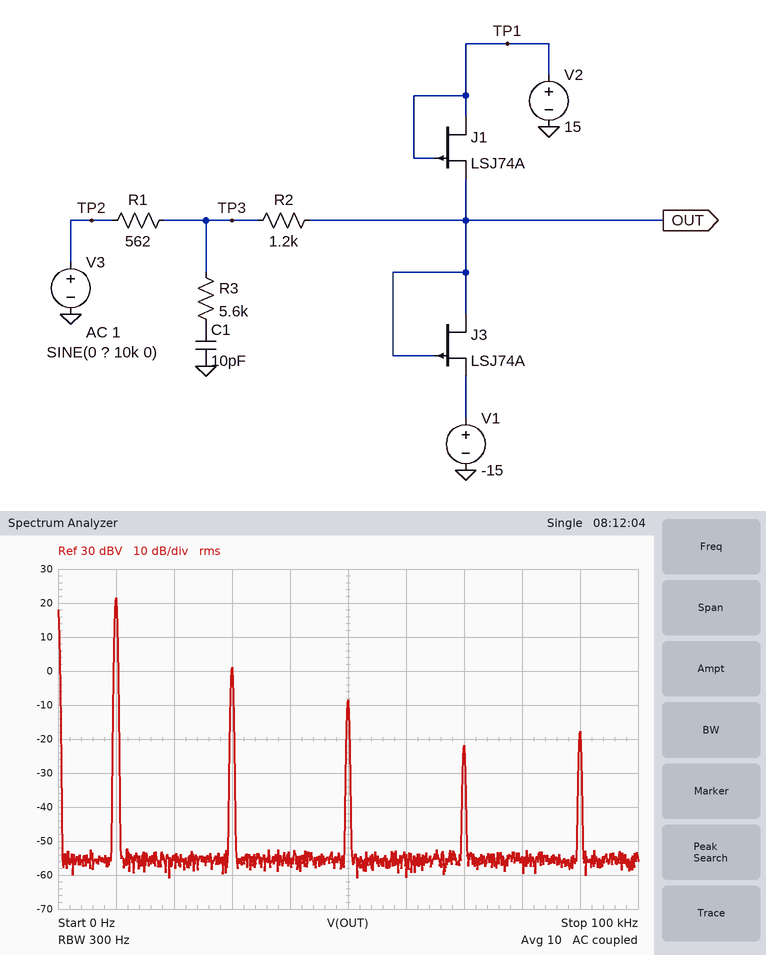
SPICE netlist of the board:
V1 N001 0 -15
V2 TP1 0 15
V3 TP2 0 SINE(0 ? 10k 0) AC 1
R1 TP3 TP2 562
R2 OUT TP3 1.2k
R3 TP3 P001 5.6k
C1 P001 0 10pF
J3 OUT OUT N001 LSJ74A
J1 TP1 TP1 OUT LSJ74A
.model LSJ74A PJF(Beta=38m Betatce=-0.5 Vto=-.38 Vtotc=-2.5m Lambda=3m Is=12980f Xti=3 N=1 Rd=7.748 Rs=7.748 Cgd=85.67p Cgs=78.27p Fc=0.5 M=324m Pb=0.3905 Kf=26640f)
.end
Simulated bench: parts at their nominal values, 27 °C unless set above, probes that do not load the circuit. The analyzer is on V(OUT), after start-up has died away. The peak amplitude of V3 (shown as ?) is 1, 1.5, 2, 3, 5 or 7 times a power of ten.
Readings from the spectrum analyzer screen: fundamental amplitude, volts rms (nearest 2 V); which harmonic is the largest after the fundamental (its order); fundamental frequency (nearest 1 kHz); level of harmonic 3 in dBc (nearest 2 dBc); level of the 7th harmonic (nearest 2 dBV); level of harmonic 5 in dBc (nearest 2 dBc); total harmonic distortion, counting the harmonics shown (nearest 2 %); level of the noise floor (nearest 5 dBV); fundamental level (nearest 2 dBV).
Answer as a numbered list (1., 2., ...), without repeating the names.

1. 12 V
2. 3
3. 10 kHz
4. -20 dBc
5. -22 dBV
6. -30 dBc
7. 10 %
8. -55 dBV
9. 22 dBV
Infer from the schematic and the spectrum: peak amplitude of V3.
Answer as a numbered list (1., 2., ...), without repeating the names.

1. 20 V
